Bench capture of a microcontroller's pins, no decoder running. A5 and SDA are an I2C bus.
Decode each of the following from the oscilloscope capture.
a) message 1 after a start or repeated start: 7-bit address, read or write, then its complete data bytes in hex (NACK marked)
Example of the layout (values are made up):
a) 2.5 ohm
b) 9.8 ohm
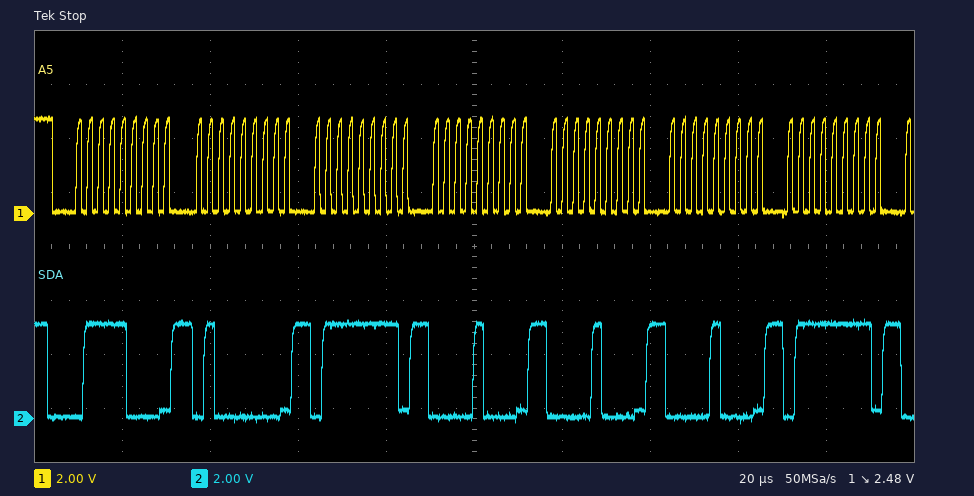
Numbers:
a) 0x3C write: 40 7F 08 08 08 7F
